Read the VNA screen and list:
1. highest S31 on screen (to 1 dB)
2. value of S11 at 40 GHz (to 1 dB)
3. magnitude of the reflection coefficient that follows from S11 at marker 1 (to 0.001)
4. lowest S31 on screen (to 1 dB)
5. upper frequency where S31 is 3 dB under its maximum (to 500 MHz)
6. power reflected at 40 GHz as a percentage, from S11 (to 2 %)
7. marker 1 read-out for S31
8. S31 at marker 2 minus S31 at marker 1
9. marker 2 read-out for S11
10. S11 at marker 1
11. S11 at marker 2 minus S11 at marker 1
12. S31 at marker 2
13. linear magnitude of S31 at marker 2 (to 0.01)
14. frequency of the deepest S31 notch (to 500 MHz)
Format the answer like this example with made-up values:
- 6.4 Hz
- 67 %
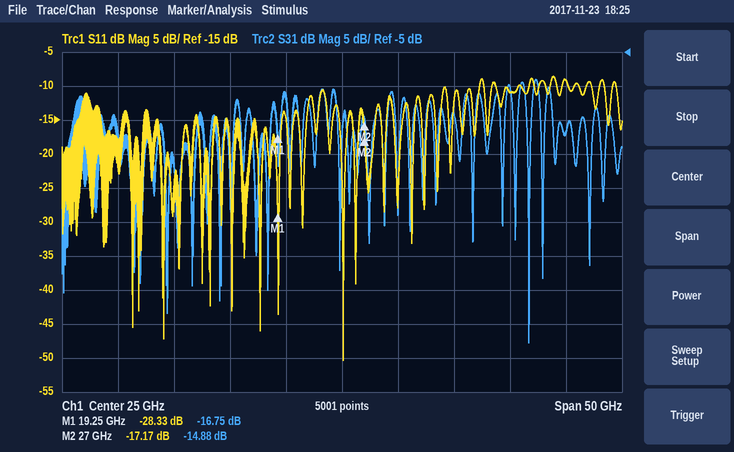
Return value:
- -9 dB
- -11 dB
- 0.038
- -48 dB
- 42.5 GHz
- 8 %
- -16.75 dB
- 1.87 dB
- -17.17 dB
- -28.33 dB
- 11.16 dB
- -14.88 dB
- 0.18
- 41.5 GHz
